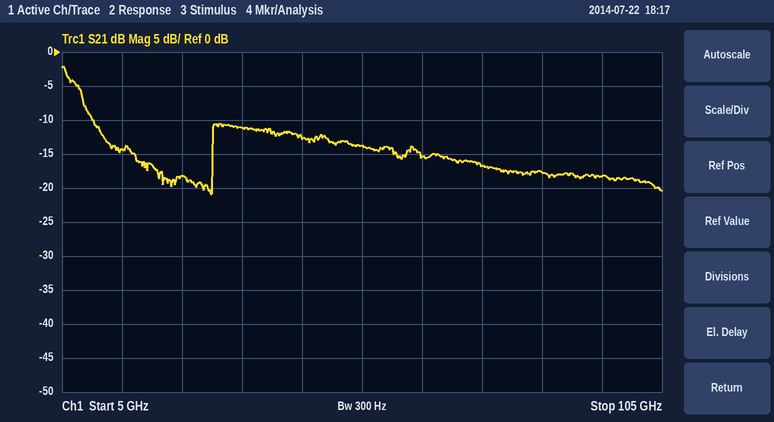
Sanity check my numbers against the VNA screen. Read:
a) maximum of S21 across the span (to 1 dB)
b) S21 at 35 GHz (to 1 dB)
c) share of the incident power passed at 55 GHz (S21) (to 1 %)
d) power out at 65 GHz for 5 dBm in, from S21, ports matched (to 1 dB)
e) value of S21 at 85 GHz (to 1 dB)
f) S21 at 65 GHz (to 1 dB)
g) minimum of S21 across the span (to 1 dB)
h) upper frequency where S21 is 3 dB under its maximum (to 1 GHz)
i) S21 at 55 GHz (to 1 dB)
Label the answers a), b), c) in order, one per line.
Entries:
a) -2 dB
b) -11 dB
c) 4 %
d) -10 dBm
e) -18 dB
f) -15 dB
g) -21 dB
h) 8 GHz
i) -14 dB
